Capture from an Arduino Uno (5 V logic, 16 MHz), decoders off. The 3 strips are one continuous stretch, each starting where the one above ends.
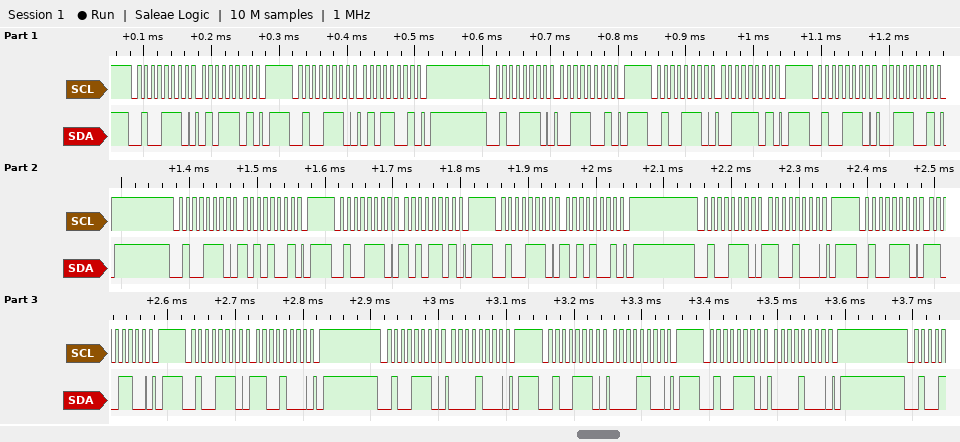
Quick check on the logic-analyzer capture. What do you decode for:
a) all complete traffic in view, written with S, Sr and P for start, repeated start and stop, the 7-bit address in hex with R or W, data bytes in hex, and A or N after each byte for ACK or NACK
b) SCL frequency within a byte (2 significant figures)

S 27W A 5D A P S 27W A 59 A P S 27W A 39 A P S 27W A 3D A P S 27W A 39 A P S 27W A A9 A P S 27W A AD A P S 27W A A9 A P S 27W A C8 A P S 27W A CC A P S 27W A C8 A P S 27W A 08 A P S 27W A 0C A P S 27W A 08 A P
100 kHz
